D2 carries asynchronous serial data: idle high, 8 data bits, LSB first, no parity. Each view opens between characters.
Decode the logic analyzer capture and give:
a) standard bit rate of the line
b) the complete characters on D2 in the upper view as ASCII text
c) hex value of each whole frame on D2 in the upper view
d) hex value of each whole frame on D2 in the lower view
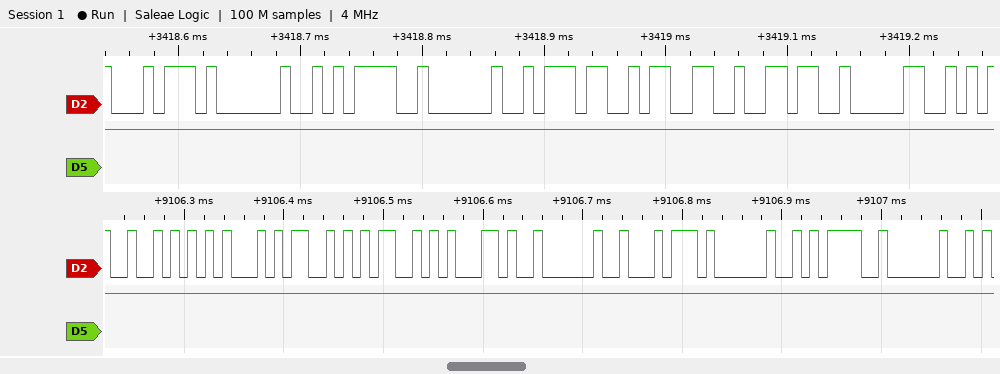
115200 baud
"t = 7360"
74, 20, 3D, 20, 37, 33, 36, 30
52, 45, 53, 53, 2C, 20, 74, 20, 3D, 20
